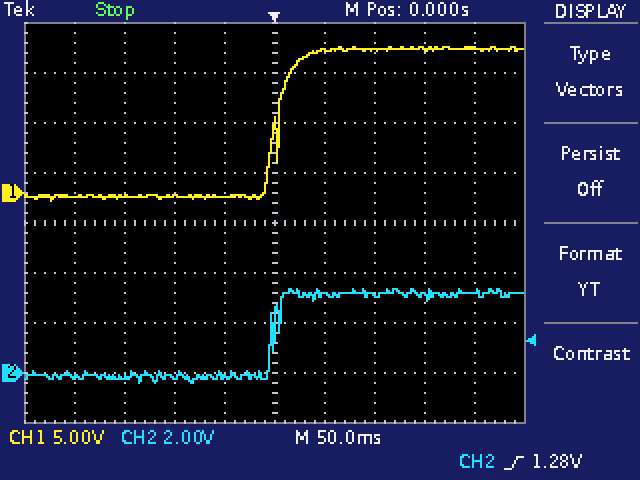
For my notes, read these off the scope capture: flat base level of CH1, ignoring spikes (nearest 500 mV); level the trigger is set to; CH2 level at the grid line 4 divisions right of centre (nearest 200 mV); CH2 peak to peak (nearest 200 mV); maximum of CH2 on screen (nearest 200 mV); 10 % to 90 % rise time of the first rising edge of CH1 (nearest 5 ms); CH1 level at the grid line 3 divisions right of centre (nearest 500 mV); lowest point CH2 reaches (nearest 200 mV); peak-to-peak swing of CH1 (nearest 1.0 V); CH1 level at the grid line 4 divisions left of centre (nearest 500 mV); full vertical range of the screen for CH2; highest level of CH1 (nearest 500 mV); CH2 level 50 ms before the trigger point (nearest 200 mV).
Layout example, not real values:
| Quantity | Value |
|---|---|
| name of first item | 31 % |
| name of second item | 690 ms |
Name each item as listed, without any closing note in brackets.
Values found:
| Quantity | Value |
|---|---|
| flat base level of CH1, ignoring spikes | -500 mV |
| level the trigger is set to | 1.28 V |
| CH2 level at the grid line 4 divisions right of centre | 3.2 V |
| CH2 peak to peak | 3.8 V |
| maximum of CH2 on screen | 3.4 V |
| 10 % to 90 % rise time of the first rising edge of CH1 | 30 ms |
| CH1 level at the grid line 3 divisions right of centre | 14.5 V |
| lowest point CH2 reaches | -400 mV |
| peak-to-peak swing of CH1 | 15.0 V |
| CH1 level at the grid line 4 divisions left of centre | -500 mV |
| full vertical range of the screen for CH2 | 16 V |
| highest level of CH1 | 14.5 V |
| CH2 level 50 ms before the trigger point | -200 mV |
